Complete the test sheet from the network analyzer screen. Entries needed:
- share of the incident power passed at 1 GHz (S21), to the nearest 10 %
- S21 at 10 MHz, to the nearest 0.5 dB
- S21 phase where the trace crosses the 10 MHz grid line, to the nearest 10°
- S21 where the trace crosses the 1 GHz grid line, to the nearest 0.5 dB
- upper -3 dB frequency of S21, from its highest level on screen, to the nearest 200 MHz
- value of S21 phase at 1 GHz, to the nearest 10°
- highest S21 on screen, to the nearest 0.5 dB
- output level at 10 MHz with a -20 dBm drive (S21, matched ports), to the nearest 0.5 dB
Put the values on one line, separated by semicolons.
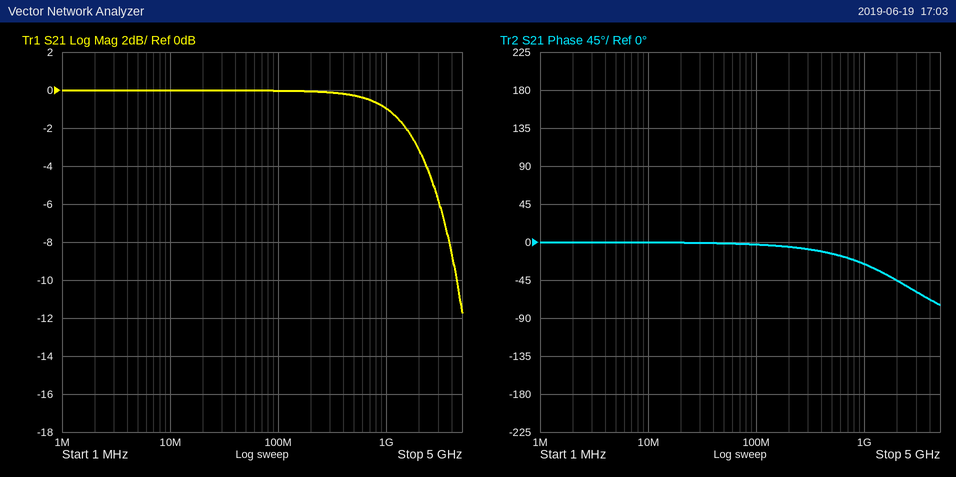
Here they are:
80 %; 0.0 dB; 0°; -1.0 dB; 2.0 GHz; -30°; 0.0 dB; -20.0 dBm
